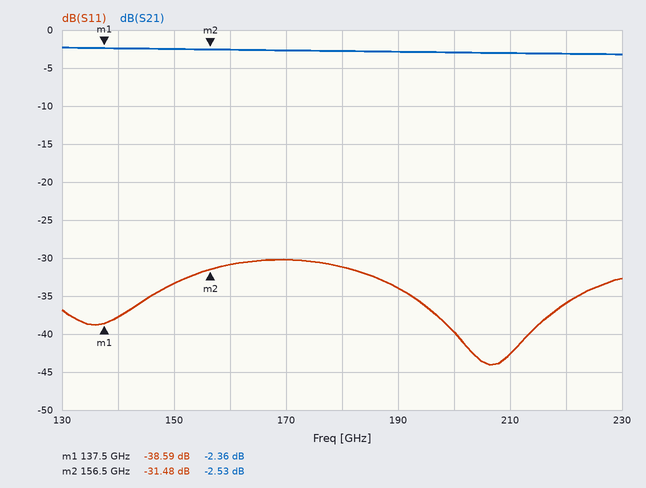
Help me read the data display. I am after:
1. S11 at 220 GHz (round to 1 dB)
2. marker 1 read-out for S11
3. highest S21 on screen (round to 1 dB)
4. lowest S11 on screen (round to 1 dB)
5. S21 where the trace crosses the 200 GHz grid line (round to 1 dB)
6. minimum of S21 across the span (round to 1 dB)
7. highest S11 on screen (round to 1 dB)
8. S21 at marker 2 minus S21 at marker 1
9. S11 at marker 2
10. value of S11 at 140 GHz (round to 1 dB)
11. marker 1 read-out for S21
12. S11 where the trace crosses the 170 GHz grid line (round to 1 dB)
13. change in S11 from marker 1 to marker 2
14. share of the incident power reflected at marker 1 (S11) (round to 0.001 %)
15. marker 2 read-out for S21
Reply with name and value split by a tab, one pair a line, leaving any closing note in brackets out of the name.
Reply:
S11 at 220 GHz	-36 dB
marker 1 read-out for S11	-38.59 dB
highest S21 on screen	-2 dB
lowest S11 on screen	-44 dB
S21 where the trace crosses the 200 GHz grid line	-3 dB
minimum of S21 across the span	-3 dB
highest S11 on screen	-30 dB
S21 at marker 2 minus S21 at marker 1	-0.17 dB
S11 at marker 2	-31.48 dB
value of S11 at 140 GHz	-38 dB
marker 1 read-out for S21	-2.36 dB
S11 where the trace crosses the 170 GHz grid line	-30 dB
change in S11 from marker 1 to marker 2	7.11 dB
share of the incident power reflected at marker 1 (S11)	0.014 %
marker 2 read-out for S21	-2.53 dB
